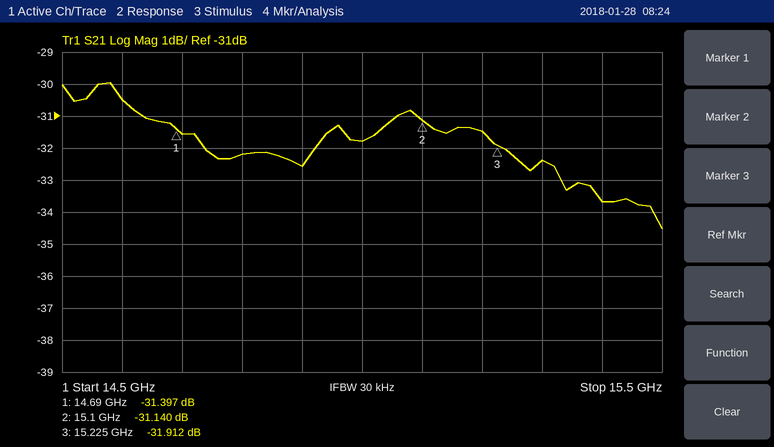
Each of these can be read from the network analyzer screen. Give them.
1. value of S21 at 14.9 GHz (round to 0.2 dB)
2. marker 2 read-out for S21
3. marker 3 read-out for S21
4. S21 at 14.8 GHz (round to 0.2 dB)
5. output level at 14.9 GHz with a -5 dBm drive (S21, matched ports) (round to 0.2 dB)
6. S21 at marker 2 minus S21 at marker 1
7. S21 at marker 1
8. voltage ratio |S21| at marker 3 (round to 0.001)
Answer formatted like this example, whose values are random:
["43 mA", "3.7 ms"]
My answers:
["-32.6 dB", "-31.140 dB", "-31.912 dB", "-32.2 dB", "-37.6 dBm", "0.257 dB", "-31.397 dB", "0.025"]
